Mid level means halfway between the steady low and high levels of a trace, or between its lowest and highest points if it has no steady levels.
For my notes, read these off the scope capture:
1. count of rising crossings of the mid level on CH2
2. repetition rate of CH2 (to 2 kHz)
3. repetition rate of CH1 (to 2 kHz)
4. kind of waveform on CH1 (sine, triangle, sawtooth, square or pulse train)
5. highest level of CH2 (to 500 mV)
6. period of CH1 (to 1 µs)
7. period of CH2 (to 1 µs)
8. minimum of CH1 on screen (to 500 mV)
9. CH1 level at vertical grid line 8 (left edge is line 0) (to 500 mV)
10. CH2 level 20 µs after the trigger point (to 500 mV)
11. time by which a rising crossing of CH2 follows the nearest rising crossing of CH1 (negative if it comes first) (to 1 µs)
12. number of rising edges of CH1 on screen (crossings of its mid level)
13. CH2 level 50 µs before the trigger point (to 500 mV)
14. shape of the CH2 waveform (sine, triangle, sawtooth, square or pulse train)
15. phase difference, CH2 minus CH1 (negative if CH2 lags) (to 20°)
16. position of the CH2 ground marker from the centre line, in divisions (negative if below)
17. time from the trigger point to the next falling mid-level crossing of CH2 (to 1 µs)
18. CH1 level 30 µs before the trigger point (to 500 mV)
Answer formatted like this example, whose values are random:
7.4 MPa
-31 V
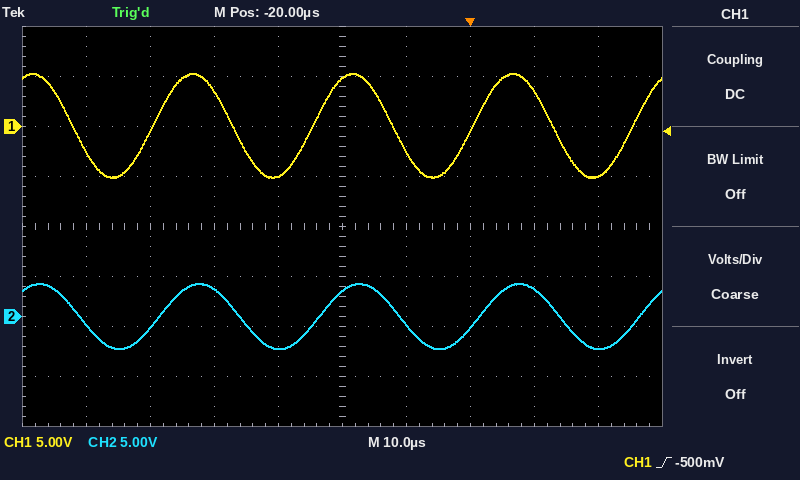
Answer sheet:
4
40 kHz
40 kHz
sine
3.5 V
25 µs
25 µs
-5.0 V
3.5 V
-3.0 V
+1 µs
4
-1.0 V
sine
-20°
-1.8 div
14 µs
-5.0 V
